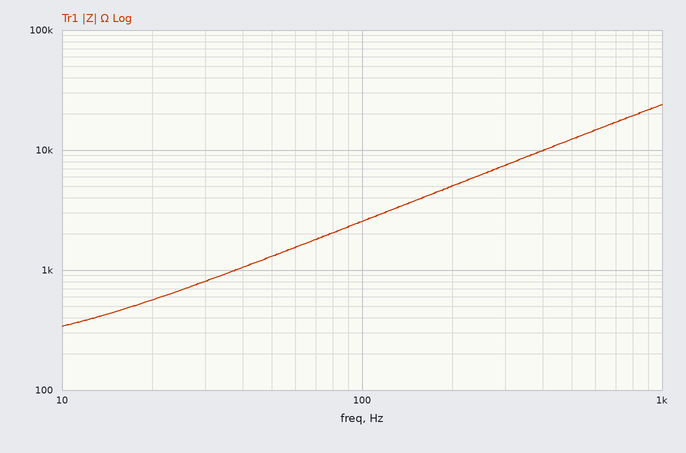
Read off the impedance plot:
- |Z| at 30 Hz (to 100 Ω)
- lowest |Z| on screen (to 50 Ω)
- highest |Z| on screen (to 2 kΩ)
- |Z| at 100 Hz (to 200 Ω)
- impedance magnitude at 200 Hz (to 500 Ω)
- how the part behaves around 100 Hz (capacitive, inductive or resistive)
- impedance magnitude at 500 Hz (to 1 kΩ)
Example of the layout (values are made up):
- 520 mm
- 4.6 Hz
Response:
- 800 Ω
- 350 Ω
- 24 kΩ
- 2.6 kΩ
- 5.0 kΩ
- inductive
- 12 kΩ
